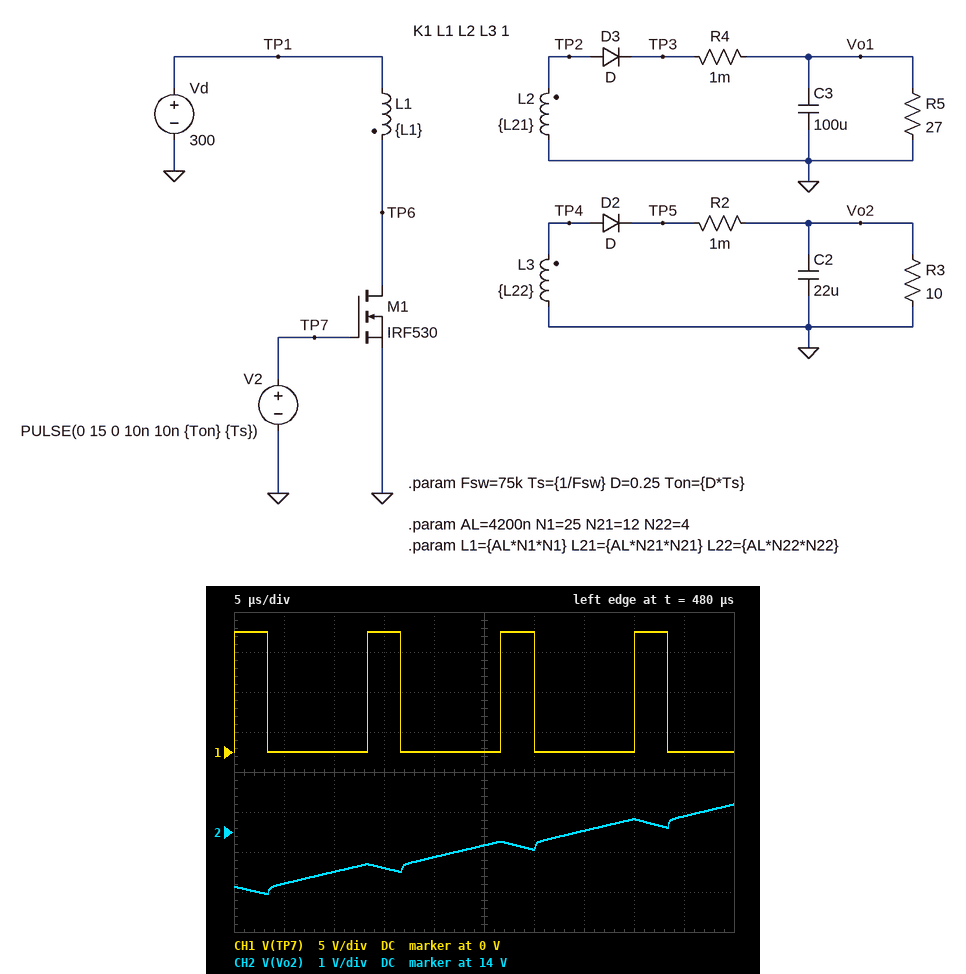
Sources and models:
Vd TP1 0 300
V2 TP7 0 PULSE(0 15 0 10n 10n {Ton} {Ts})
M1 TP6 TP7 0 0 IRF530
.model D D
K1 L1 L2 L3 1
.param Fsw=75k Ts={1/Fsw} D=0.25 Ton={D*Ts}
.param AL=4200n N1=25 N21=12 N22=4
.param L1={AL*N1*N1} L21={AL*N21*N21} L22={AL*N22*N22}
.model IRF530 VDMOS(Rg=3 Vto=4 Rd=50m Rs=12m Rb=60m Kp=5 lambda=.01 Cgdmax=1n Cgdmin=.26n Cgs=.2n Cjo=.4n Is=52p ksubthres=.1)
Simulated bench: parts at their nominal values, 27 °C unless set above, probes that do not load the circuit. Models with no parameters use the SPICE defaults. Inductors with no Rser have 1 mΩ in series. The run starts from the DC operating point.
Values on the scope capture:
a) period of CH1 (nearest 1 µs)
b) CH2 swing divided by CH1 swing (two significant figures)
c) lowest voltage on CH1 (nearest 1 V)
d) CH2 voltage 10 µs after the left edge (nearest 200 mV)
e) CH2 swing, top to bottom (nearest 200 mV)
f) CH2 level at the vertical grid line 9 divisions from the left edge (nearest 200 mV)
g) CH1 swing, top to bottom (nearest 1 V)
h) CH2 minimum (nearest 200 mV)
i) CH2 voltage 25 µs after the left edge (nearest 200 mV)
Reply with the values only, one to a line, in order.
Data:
13 µs
0.15
0 V
13.0 V
2.2 V
14.4 V
15 V
12.4 V
13.6 V
